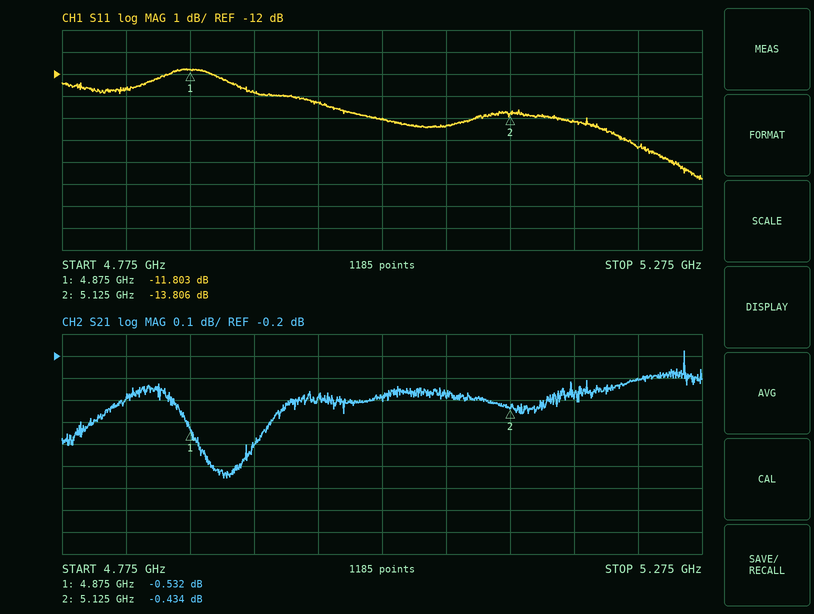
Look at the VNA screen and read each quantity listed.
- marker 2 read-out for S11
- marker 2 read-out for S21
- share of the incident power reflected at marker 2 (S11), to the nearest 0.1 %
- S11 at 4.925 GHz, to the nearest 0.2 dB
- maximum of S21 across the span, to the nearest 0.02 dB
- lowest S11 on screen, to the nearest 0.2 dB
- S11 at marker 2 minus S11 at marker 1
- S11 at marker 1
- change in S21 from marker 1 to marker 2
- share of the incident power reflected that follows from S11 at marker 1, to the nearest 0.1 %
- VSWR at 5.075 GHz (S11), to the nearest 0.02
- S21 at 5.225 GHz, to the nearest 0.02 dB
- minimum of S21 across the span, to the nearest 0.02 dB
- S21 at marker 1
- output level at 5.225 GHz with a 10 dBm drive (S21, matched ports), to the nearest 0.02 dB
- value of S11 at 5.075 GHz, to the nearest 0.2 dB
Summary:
-13.806 dB
-0.434 dB
4.2 %
-12.8 dB
-0.18 dB
-16.8 dB
-2.003 dB
-11.803 dB
0.098 dB
6.6 %
1.48
-0.30 dB
-0.76 dB
-0.532 dB
9.70 dBm
-14.4 dB
